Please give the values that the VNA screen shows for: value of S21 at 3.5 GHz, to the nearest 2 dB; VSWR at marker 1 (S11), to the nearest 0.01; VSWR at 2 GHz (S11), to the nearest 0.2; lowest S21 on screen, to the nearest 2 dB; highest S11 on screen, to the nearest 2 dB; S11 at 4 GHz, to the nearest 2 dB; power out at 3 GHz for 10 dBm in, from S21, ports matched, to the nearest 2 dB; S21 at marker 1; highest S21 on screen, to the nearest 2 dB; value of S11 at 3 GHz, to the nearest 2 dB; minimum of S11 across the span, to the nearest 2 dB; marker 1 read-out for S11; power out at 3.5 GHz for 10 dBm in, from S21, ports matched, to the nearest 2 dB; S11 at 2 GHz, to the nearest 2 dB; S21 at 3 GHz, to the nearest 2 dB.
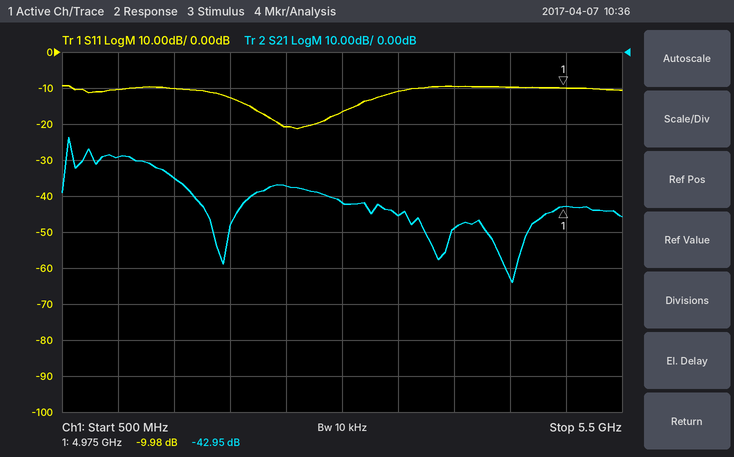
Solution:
-46 dB
1.93
1.6
-64 dB
-10 dB
-10 dB
-32 dBm
-42.95 dB
-24 dB
-16 dB
-22 dB
-9.98 dB
-36 dBm
-12 dB
-42 dB
